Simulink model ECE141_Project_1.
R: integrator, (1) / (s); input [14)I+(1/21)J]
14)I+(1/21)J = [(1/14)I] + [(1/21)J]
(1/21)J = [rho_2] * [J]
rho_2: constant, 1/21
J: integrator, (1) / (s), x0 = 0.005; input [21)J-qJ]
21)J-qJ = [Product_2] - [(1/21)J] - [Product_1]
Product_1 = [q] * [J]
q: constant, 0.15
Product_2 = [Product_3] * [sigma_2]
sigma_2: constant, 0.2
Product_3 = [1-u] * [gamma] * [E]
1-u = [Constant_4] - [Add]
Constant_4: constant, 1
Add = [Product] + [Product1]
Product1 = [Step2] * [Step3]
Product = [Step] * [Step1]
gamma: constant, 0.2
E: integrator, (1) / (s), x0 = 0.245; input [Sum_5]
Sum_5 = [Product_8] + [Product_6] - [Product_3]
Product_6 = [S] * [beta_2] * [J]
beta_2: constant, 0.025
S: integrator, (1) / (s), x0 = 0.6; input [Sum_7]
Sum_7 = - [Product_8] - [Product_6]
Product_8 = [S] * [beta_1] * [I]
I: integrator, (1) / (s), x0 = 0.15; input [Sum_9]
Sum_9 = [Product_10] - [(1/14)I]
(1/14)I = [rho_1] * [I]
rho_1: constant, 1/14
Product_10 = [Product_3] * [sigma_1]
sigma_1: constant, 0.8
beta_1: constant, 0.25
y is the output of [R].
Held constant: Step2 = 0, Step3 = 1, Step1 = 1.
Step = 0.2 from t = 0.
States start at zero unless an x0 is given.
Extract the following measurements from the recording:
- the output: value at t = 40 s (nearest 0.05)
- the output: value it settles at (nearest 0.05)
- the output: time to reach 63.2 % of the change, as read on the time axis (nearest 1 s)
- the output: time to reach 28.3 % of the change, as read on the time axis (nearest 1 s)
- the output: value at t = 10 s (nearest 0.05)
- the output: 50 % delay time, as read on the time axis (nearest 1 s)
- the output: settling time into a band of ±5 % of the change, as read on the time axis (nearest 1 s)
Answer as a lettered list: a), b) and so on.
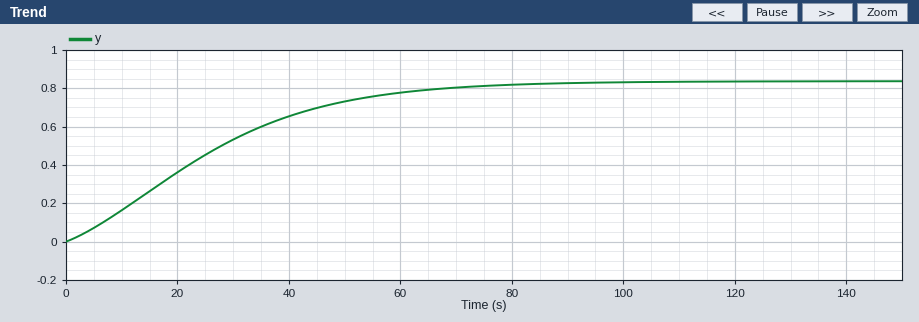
a) 0.65
b) 0.85
c) 30 s
d) 14 s
e) 0.15
f) 23 s
g) 66 s
